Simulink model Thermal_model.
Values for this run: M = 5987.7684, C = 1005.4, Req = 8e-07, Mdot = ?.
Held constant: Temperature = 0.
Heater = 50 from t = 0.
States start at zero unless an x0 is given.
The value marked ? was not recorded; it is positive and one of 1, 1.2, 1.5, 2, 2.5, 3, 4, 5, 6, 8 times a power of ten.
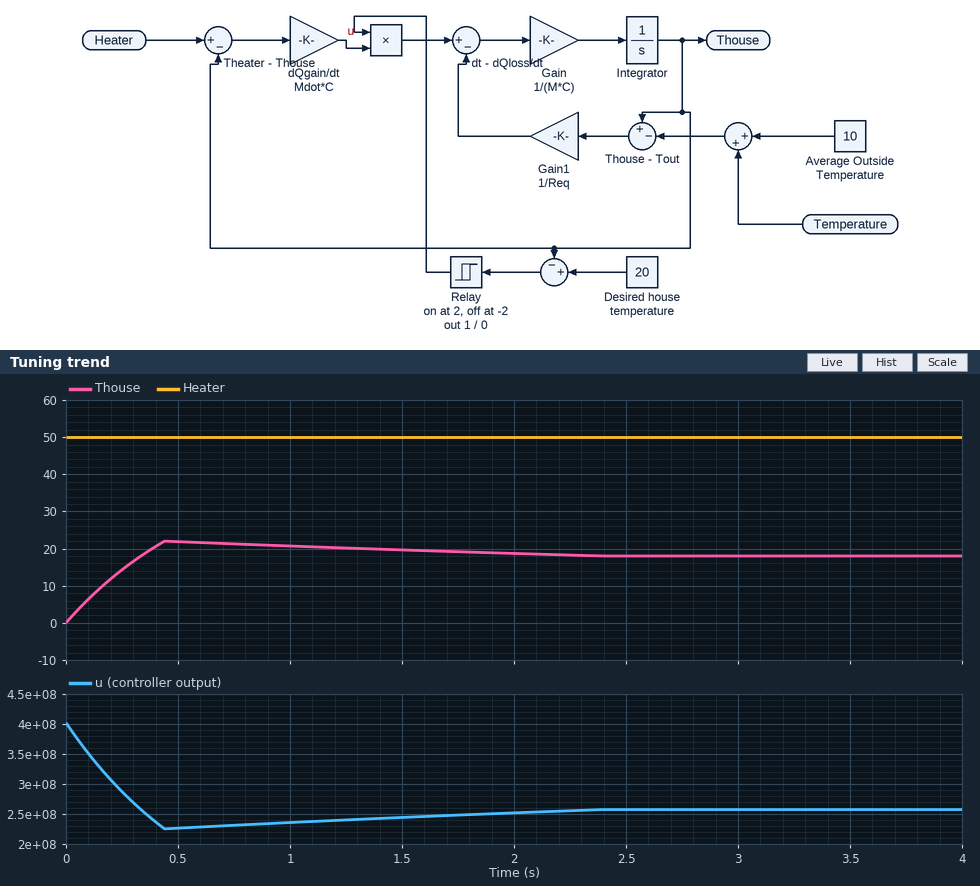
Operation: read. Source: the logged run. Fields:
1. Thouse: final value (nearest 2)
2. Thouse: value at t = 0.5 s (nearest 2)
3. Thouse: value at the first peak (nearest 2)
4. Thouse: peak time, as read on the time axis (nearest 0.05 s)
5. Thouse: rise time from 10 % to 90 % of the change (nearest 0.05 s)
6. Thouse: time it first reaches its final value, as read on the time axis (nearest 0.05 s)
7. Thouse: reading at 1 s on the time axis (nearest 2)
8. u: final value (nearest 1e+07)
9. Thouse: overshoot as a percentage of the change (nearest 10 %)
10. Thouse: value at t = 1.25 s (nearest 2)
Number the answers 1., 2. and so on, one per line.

1. 18
2. 22
3. 22
4. 0.45 s
5. 0.25 s
6. 0.35 s
7. 20
8. 260000000
9. 20 %
10. 20
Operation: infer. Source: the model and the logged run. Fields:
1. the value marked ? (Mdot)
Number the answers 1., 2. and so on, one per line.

1. 8000
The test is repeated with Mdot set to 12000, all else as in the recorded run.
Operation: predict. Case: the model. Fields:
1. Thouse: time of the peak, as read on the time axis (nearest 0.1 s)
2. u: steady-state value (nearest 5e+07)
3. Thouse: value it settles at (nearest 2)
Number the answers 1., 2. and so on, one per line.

1. 0.3 s
2. 400000000
3. 18
